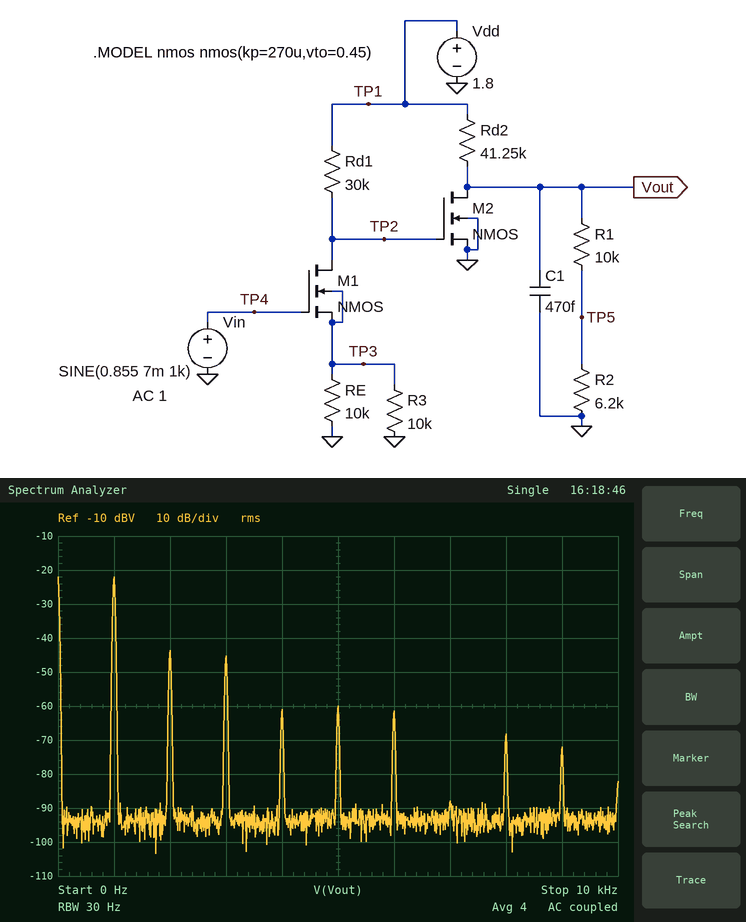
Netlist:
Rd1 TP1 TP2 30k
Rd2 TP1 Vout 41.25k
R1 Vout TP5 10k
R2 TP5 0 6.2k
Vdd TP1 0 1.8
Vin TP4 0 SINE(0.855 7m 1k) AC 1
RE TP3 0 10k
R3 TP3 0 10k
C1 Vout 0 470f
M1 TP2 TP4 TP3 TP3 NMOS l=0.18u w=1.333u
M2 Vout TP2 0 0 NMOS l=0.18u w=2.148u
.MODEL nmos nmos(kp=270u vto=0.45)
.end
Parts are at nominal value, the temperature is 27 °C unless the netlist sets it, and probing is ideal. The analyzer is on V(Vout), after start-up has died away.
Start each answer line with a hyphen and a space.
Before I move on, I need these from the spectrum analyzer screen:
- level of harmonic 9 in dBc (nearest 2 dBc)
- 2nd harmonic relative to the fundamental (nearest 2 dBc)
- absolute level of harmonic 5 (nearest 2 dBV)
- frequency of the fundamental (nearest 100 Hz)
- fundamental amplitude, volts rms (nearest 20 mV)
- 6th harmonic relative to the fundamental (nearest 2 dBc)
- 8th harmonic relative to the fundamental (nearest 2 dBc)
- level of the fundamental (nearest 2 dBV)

- -50 dBc
- -22 dBc
- -60 dBV
- 1.0 kHz
- 80 mV
- -40 dBc
- -46 dBc
- -22 dBV
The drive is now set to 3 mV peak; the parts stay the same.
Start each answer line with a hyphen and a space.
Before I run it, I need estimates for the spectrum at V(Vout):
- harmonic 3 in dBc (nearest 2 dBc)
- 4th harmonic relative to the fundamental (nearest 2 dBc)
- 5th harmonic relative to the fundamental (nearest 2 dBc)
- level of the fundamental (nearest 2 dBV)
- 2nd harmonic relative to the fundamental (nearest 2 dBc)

- -44 dBc
- -46 dBc
- -48 dBc
- -28 dBV
- -36 dBc
